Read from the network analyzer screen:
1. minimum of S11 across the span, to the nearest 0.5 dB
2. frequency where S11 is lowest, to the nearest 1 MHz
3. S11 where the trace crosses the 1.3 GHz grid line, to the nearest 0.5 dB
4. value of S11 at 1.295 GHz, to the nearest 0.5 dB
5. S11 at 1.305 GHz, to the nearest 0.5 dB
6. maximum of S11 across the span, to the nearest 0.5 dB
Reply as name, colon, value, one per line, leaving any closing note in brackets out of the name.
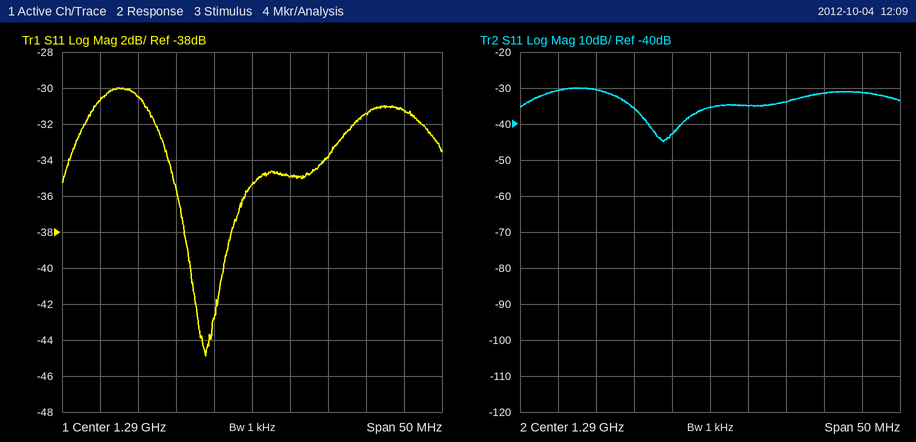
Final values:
minimum of S11 across the span, to the nearest 0.5 dB: -45.0 dB
frequency where S11 is lowest, to the nearest 1 MHz: 1.284 GHz
S11 where the trace crosses the 1.3 GHz grid line, to the nearest 0.5 dB: -34.0 dB
value of S11 at 1.295 GHz, to the nearest 0.5 dB: -35.0 dB
S11 at 1.305 GHz, to the nearest 0.5 dB: -31.5 dB
maximum of S11 across the span, to the nearest 0.5 dB: -30.0 dB
